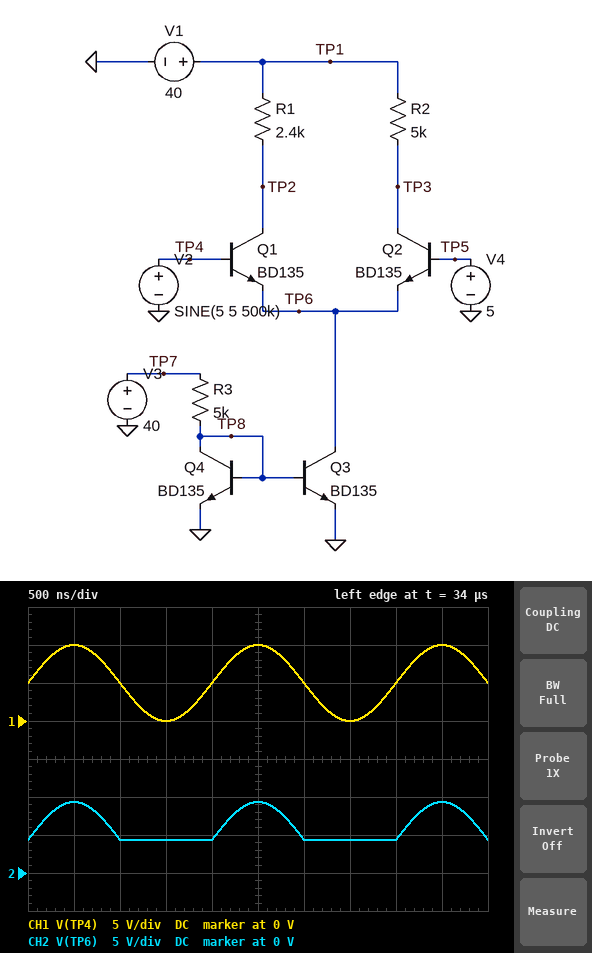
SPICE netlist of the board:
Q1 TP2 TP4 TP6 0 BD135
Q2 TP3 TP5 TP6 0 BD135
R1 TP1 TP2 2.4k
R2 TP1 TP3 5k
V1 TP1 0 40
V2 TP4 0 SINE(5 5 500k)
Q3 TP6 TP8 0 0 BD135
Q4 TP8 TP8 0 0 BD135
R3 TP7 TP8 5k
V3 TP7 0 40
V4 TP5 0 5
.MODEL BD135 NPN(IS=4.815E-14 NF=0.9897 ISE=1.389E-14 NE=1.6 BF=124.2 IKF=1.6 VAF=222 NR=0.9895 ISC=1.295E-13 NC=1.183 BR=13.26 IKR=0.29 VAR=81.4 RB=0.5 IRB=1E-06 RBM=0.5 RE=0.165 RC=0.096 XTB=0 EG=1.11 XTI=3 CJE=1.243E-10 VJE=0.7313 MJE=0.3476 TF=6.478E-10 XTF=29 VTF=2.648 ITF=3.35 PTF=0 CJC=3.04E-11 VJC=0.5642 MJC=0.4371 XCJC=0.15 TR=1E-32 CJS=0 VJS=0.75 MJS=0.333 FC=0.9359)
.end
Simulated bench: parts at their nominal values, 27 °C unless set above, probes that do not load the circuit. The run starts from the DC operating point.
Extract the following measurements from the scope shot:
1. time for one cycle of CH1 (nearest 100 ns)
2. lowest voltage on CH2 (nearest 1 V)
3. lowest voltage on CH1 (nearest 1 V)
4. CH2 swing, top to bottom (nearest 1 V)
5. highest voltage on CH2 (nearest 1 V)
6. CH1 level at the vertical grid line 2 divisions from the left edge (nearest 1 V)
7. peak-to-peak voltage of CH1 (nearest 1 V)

2.0 µs
4 V
0 V
5 V
9 V
5 V
10 V
